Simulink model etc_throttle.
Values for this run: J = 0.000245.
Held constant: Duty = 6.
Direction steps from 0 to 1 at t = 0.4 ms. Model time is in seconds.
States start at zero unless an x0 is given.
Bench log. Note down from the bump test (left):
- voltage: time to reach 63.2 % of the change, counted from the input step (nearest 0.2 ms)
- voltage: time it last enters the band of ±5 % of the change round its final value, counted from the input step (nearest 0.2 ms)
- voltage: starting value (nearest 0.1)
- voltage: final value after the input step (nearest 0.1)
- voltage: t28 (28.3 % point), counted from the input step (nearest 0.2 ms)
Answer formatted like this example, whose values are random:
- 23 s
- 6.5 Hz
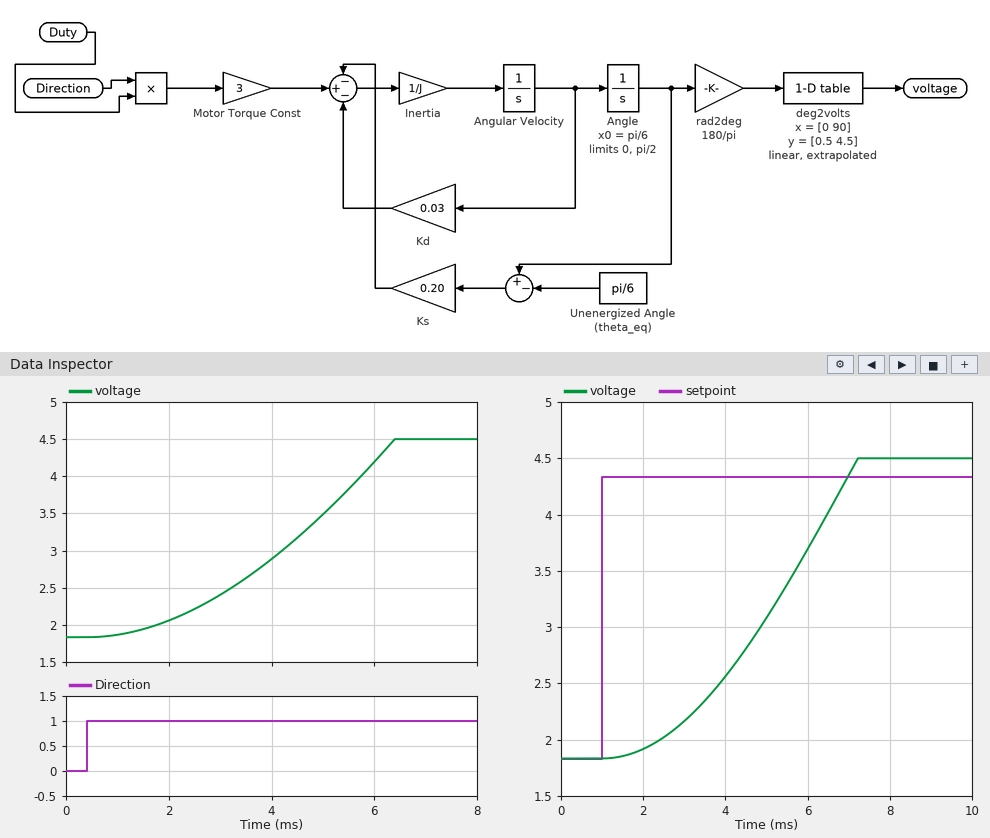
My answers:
- 4.6 ms
- 5.8 ms
- 1.8
- 4.5
- 3.0 ms
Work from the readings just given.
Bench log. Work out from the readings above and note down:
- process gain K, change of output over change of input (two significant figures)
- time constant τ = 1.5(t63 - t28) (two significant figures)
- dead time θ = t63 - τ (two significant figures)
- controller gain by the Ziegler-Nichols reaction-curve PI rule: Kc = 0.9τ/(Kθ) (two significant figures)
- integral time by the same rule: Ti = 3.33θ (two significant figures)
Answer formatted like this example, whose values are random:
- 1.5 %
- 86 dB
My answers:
- 2.7
- 2.4 ms
- 2.2 ms
- 0.36
- 7.3 ms
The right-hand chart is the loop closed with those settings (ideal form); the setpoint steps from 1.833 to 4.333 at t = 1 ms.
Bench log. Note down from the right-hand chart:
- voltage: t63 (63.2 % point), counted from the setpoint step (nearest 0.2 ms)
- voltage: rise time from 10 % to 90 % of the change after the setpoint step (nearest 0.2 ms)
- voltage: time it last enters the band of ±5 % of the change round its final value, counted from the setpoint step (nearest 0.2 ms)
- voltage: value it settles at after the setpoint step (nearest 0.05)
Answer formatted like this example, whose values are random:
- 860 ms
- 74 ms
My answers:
- 4.8 ms
- 4.0 ms
- 6.0 ms
- 4.50
